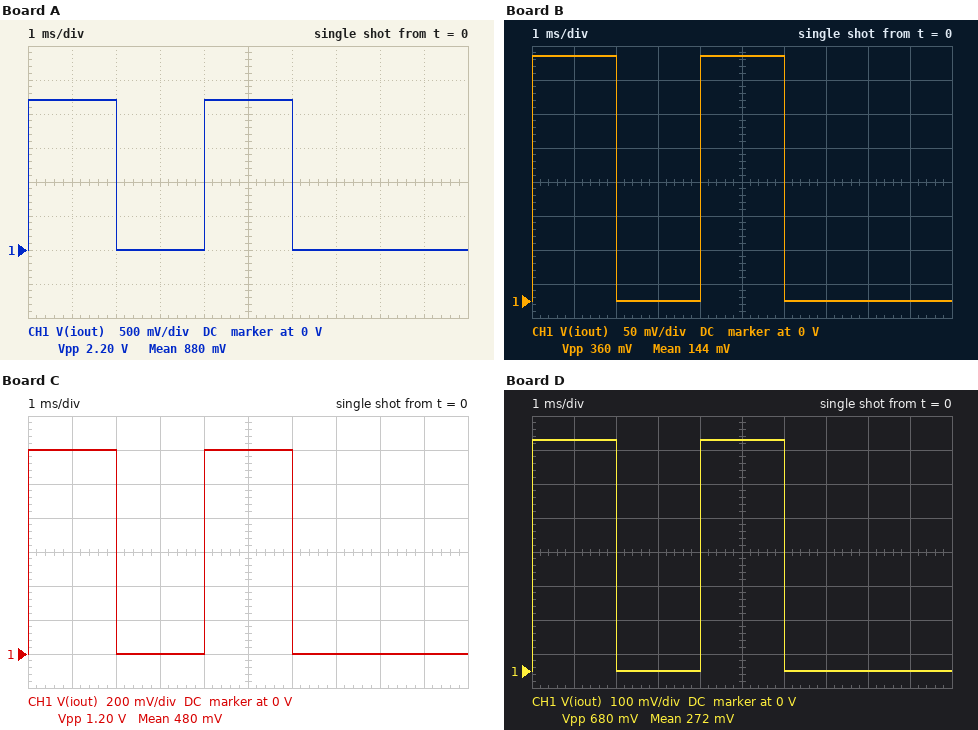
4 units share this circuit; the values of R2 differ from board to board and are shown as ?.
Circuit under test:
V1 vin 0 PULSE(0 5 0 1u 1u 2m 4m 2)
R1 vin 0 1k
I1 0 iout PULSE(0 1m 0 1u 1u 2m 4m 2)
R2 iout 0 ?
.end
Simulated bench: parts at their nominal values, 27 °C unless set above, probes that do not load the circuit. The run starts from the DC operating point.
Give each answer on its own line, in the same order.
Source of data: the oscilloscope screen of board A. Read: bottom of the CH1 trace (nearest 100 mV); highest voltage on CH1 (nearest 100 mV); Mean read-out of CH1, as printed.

0 V
2.2 V
880 mV
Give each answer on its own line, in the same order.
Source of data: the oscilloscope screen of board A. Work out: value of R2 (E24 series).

2.2 kΩ
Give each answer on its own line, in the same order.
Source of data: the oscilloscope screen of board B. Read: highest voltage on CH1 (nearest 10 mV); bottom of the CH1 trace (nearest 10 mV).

360 mV
0 V
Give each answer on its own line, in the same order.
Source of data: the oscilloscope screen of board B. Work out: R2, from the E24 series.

360 Ω
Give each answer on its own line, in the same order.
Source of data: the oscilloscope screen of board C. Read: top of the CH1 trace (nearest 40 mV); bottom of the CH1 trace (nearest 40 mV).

1.20 V
0 V
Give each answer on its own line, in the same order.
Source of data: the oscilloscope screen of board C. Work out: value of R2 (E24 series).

1.2 kΩ
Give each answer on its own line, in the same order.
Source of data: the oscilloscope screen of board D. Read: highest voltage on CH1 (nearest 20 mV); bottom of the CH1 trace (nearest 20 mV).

680 mV
0 V
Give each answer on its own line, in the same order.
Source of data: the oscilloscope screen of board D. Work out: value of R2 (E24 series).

680 Ω
